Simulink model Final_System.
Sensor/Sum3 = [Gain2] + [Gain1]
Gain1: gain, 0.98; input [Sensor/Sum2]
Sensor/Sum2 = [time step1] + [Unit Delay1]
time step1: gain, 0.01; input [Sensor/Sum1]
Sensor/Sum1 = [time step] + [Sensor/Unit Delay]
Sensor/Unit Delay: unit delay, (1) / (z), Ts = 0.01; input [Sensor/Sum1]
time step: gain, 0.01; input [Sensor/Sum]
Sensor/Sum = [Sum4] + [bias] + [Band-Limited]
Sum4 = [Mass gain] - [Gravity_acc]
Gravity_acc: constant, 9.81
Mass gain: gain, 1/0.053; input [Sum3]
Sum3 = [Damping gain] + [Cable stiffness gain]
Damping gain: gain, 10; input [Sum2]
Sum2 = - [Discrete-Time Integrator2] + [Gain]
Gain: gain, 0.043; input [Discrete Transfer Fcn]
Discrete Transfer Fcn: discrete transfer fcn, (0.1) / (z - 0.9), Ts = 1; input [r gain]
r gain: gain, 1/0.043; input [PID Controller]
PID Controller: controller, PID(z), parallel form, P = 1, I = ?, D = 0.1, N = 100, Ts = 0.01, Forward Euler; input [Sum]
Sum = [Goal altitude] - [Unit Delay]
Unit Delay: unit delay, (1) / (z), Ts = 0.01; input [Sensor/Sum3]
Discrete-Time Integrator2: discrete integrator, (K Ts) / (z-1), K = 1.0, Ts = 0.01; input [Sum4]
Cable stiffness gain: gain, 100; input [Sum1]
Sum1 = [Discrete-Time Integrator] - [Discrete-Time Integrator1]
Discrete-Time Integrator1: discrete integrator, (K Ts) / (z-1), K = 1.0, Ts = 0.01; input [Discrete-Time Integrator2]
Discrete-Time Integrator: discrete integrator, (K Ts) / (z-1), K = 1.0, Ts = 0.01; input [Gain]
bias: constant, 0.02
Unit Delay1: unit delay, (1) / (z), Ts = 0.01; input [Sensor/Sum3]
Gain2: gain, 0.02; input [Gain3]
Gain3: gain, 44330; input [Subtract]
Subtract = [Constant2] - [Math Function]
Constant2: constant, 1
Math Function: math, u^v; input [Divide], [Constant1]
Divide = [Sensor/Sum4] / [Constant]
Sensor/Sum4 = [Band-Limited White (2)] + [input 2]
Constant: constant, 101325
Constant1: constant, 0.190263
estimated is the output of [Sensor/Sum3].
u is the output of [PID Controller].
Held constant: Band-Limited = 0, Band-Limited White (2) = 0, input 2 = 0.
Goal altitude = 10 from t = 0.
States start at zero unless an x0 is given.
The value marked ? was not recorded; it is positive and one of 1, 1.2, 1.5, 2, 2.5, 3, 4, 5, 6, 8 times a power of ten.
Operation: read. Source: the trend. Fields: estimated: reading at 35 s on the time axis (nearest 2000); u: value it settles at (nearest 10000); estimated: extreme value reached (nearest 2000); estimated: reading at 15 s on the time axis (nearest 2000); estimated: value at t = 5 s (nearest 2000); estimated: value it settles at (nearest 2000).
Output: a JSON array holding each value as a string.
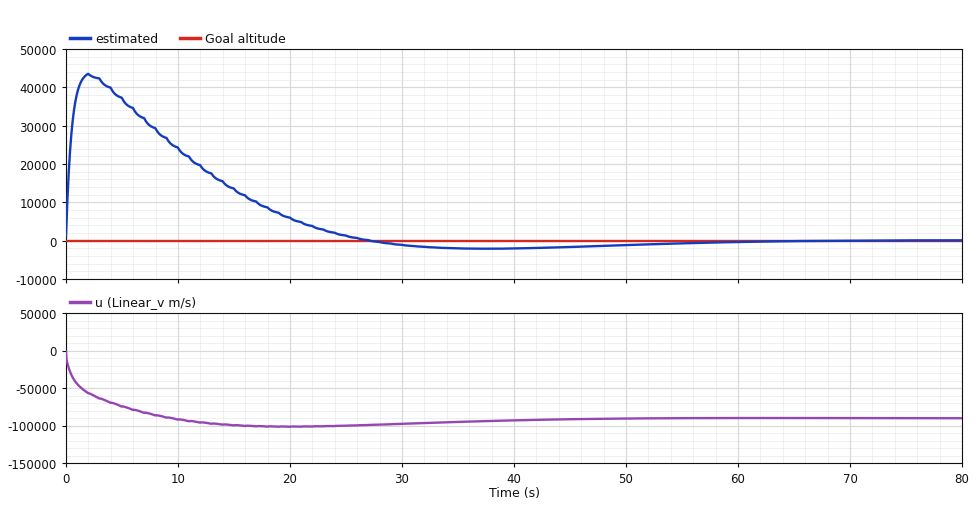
["-2000", "-90000", "44000", "14000", "38000", "0"]
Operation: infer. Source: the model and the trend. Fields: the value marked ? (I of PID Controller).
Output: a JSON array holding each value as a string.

["0.2"]
